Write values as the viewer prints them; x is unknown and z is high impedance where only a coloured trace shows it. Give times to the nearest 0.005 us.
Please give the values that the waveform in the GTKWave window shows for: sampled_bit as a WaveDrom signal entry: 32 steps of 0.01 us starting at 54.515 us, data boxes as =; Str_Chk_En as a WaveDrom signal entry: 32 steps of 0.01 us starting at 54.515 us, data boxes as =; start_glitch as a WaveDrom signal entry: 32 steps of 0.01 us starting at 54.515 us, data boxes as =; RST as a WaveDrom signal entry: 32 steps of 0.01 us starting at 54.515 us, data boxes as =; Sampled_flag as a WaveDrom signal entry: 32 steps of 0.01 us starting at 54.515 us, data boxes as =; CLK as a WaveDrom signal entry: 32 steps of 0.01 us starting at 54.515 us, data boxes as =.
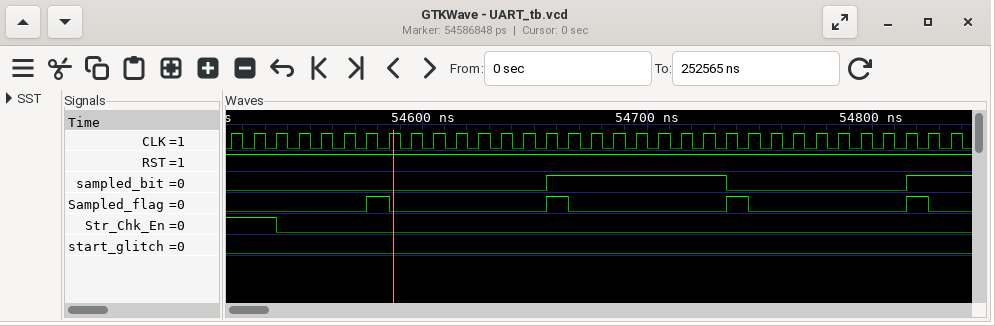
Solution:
{name: 'sampled_bit', wave: '0.............1.......0.......1.'}
{name: 'Str_Chk_En', wave: '1.0.............................'}
{name: 'start_glitch', wave: '0...............................'}
{name: 'RST', wave: '1...............................'}
{name: 'Sampled_flag', wave: '0.....10......10......10......10'}
{name: 'CLK', wave: 'p...............................'}
